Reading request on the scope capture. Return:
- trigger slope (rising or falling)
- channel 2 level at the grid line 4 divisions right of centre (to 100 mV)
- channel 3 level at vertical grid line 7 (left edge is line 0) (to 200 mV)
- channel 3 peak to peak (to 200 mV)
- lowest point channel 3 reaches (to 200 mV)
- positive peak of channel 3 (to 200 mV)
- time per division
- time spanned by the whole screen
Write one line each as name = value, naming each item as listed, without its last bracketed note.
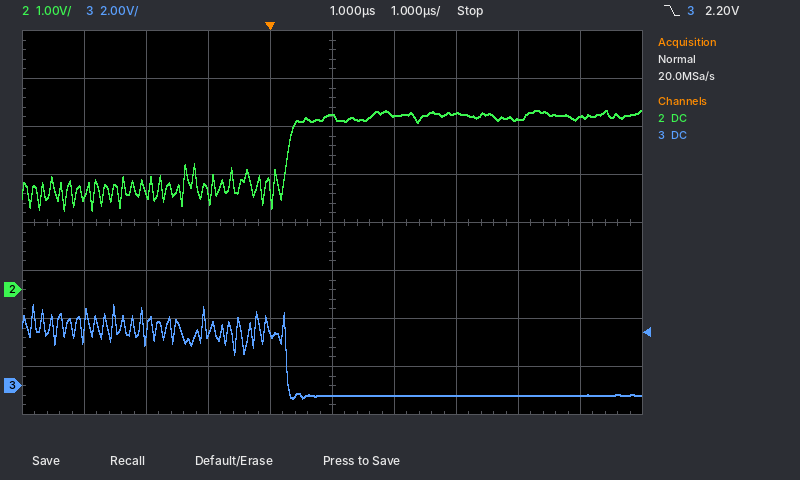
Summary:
trigger slope = falling
channel 2 level at the grid line 4 divisions right of centre = 3.6 V
channel 3 level at vertical grid line 7 (left edge is line 0) = -400 mV
channel 3 peak to peak = 4.0 V
lowest point channel 3 reaches = -600 mV
positive peak of channel 3 = 3.4 V
time per division = 1 µs
time spanned by the whole screen = 10 µs
